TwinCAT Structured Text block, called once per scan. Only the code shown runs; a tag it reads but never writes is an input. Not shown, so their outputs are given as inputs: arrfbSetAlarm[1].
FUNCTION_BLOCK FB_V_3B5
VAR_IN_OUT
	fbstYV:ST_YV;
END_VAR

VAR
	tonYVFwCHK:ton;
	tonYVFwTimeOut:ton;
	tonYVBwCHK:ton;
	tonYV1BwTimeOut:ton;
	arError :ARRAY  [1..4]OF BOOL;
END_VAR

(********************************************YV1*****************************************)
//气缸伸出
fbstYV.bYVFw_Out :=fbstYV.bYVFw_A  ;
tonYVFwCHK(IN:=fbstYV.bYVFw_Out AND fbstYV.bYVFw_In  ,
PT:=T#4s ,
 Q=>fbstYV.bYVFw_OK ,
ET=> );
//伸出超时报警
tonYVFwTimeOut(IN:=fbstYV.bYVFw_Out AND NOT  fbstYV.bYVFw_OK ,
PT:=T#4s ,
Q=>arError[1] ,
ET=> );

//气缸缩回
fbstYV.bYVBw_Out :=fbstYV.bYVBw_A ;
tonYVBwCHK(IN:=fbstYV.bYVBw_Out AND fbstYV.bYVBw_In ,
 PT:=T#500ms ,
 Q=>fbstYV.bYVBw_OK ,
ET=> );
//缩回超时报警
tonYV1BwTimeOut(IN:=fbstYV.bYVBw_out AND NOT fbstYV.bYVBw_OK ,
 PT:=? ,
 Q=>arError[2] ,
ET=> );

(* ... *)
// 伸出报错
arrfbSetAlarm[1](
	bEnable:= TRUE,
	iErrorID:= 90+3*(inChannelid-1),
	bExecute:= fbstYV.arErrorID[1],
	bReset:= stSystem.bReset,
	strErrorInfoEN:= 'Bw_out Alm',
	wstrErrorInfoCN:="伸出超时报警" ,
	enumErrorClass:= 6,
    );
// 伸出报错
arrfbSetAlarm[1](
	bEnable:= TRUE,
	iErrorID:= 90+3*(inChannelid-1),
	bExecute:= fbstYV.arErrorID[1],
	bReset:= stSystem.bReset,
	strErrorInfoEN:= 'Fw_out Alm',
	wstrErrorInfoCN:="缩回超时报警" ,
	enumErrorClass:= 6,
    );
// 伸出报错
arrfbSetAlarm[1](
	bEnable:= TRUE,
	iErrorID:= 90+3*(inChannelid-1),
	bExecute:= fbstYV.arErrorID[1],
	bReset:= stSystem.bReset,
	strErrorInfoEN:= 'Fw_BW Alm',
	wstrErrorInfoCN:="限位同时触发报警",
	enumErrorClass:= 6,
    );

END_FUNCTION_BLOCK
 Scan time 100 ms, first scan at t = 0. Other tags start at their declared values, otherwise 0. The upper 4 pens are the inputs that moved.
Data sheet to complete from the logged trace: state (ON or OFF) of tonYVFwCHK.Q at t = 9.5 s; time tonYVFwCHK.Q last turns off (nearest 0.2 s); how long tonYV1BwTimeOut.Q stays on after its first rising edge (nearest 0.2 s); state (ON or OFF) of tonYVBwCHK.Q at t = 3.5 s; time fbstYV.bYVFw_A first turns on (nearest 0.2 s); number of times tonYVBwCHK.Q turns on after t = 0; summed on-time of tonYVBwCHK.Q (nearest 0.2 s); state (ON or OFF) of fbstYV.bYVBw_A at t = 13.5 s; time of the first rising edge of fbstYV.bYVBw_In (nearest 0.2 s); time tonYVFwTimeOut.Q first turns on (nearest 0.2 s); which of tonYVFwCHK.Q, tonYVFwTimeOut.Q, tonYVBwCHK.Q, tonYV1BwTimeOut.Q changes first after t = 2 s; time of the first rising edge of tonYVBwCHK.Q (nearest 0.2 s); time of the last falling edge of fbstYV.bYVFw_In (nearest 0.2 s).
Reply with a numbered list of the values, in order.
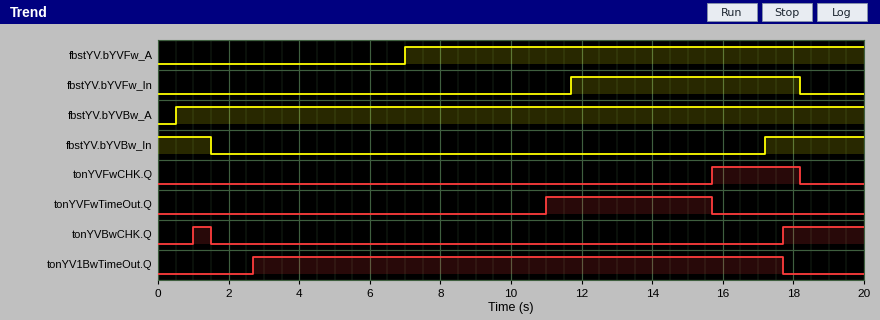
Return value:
1. OFF
2. 18.2 s
3. 15.0 s
4. OFF
5. 7.0 s
6. 2
7. 2.8 s
8. ON
9. 17.2 s
10. 11.0 s
11. tonYV1BwTimeOut.Q
12. 1.0 s
13. 18.2 s
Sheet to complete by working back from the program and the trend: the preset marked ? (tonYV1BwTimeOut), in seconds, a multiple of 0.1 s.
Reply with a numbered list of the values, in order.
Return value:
1. 1.2 s
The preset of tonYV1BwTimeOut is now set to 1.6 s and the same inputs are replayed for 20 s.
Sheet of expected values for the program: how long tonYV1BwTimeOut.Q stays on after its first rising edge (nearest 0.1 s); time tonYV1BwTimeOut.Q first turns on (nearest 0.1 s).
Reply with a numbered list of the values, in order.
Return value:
1. 14.6 s
2. 3.1 s
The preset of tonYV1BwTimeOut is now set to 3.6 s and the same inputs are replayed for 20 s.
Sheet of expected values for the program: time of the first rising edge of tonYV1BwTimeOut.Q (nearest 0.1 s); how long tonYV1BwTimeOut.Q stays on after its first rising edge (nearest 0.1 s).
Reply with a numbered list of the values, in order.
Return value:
1. 5.1 s
2. 12.6 s
